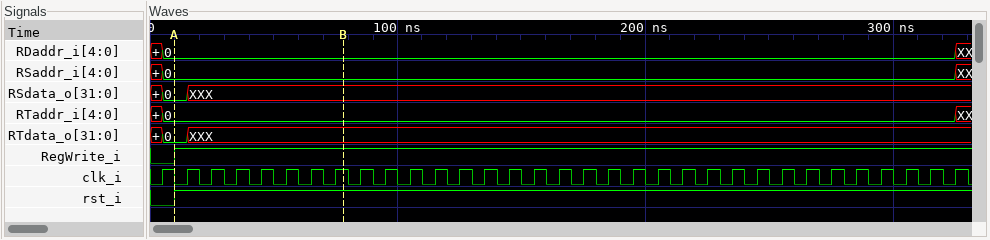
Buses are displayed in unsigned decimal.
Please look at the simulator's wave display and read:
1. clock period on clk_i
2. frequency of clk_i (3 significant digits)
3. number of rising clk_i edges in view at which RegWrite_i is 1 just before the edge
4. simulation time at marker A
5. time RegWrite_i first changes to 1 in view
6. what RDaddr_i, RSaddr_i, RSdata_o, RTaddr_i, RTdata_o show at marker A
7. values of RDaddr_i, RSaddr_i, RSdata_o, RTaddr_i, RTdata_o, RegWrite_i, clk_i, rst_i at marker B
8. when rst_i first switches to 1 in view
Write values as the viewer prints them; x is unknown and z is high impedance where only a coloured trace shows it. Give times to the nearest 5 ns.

10 ns
100 MHz
32
10 ns
10 ns
RDaddr_i=0, RSaddr_i=0, RSdata_o=0, RTaddr_i=0, RTdata_o=0
RDaddr_i=0, RSaddr_i=0, RSdata_o=XXX, RTaddr_i=0, RTdata_o=XXX, RegWrite_i=1, clk_i=1, rst_i=1
10 ns
